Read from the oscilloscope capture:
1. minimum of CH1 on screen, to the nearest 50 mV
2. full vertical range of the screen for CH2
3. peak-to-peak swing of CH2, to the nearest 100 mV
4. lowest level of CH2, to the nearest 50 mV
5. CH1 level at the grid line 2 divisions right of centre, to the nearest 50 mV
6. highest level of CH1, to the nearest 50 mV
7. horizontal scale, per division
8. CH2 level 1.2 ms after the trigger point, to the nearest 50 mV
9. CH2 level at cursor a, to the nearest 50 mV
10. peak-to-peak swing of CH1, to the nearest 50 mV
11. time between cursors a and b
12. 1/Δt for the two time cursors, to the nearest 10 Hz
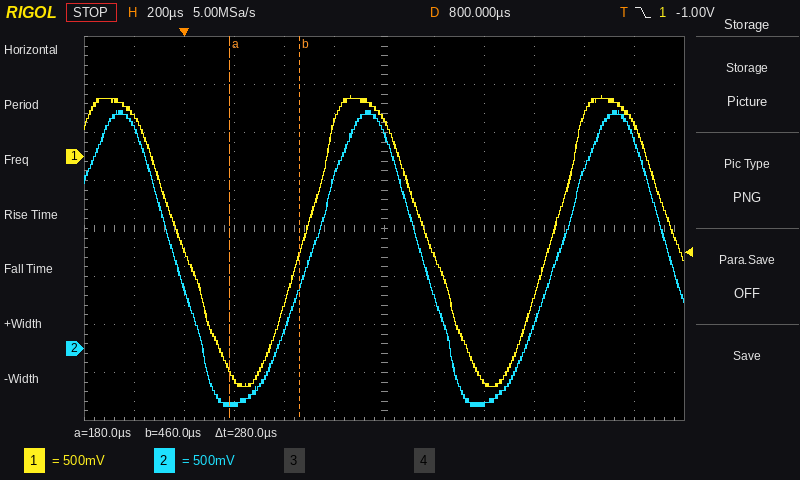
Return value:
-2.40 V
4 V
3.10 V
-600 mV
-2.35 V
650 mV
200 µs
-600 mV
-600 mV
3.05 V
280 µs
3.57 kHz
